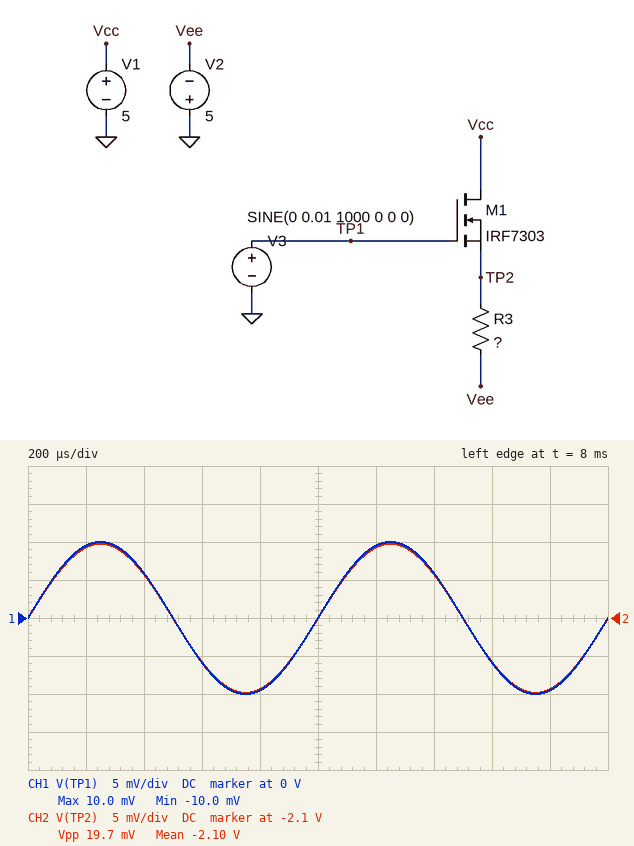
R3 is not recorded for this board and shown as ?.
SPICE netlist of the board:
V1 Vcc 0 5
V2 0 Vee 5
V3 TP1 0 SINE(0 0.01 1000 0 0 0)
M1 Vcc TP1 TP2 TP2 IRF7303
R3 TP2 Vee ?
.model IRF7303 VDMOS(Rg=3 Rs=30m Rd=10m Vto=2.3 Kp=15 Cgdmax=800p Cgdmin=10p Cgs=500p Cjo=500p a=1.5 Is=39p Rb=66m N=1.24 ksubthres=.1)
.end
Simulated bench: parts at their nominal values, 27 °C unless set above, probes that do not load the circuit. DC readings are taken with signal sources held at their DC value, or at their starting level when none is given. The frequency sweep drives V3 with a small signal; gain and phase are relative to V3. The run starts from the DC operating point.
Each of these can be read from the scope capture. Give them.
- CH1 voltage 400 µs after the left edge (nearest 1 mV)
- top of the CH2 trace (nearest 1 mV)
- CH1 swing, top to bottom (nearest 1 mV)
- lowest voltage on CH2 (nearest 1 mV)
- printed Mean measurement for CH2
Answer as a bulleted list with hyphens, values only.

- 6 mV
- -2.090 V
- 20 mV
- -2.110 V
- -2.10 V
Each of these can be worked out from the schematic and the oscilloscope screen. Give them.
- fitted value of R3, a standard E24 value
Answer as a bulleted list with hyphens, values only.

- 2.4 kΩ
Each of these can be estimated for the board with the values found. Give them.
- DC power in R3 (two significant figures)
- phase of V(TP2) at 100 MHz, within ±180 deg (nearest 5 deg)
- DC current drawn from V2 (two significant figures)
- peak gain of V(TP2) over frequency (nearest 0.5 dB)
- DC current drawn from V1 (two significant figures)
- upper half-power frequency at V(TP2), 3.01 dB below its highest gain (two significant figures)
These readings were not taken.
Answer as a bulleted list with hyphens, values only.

- 3.5 mW
- -20 deg
- 1.2 mA
- 0 dB
- 1.2 mA
- 140 MHz
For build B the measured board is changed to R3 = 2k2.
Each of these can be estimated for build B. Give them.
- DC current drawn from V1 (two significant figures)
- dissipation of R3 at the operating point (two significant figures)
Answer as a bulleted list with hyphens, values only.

- 1.3 mA
- 3.8 mW
